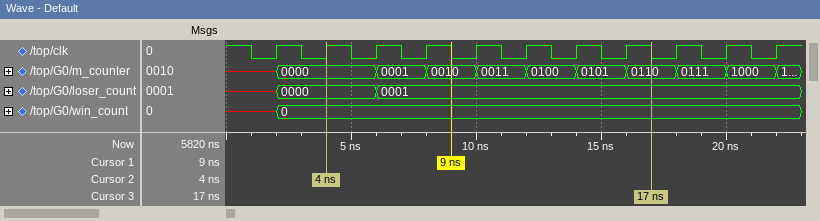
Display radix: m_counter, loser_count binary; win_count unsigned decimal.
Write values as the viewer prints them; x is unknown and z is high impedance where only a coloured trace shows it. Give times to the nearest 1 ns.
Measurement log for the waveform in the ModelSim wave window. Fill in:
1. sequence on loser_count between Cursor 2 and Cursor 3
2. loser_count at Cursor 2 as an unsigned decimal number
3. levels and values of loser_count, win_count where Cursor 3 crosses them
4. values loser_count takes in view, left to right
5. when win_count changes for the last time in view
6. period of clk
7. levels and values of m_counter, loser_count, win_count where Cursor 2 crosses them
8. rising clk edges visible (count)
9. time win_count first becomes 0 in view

0000, 0001
0
loser_count=0001, win_count=0
x, 0000, 0001
2 ns
2 ns
m_counter=0000, loser_count=0000, win_count=0
11
2 ns
